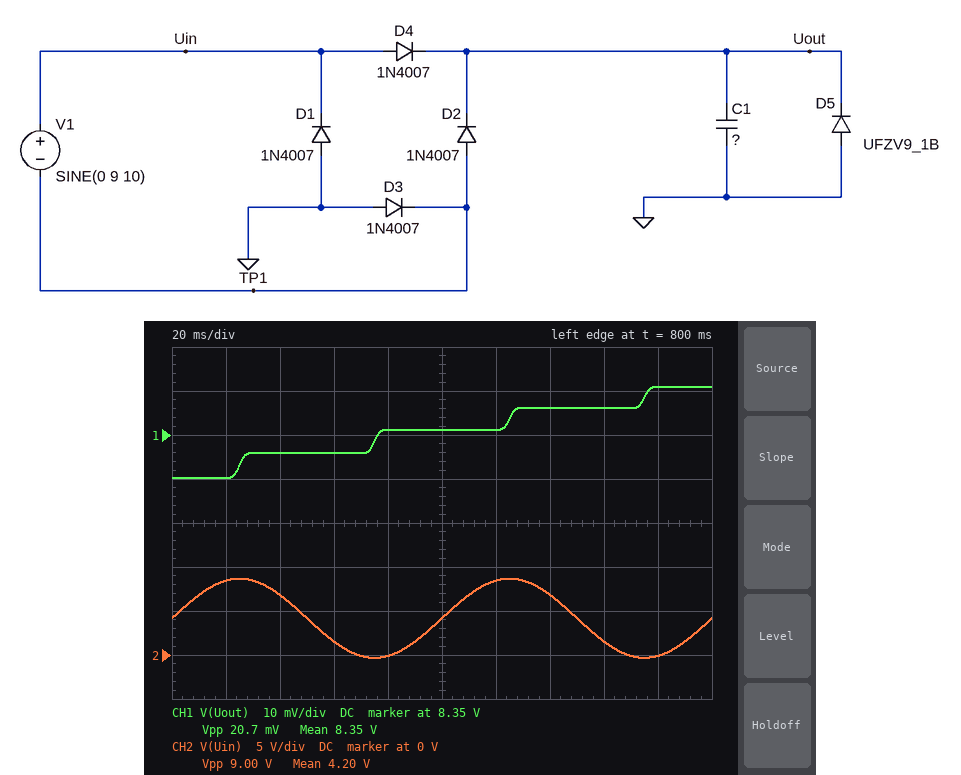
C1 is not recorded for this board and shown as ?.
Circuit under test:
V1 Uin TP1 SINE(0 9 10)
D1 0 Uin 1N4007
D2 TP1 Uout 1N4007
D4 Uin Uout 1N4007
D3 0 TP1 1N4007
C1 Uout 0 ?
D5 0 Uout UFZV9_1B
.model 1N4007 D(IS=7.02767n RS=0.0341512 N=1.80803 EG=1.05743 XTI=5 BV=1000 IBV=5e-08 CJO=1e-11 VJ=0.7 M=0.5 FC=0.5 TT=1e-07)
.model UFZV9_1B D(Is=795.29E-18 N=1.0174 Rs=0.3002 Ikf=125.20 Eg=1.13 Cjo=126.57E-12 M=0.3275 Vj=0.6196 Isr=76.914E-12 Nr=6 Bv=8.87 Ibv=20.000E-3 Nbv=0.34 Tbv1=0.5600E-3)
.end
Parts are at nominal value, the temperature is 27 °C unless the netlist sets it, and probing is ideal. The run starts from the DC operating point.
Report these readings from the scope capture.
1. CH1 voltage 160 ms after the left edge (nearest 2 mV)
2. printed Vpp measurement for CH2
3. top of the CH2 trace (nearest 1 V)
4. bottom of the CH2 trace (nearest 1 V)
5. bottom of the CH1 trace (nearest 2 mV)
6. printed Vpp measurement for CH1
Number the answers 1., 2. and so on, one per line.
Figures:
1. 8.356 V
2. 9.00 V
3. 9 V
4. 0 V
5. 8.340 V
6. 20.7 mV
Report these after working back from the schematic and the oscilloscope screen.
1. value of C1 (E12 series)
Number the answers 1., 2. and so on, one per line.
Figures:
1. 5.6 µF
